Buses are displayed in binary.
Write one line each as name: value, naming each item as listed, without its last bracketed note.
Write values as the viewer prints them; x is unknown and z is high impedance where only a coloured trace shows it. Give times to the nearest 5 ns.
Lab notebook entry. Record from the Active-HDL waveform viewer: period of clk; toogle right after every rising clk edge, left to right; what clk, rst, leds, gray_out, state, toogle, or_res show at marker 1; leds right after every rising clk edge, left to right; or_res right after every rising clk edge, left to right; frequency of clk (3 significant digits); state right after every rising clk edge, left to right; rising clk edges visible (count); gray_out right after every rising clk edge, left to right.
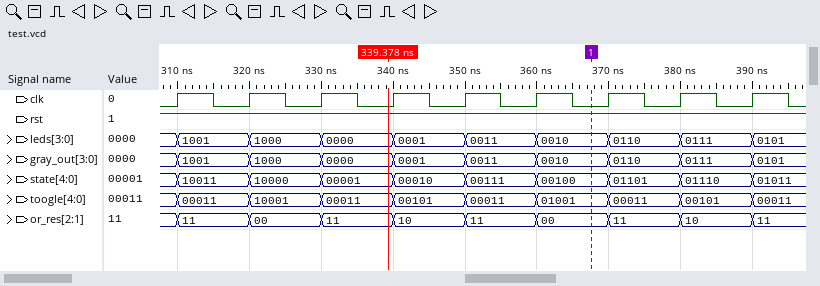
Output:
period of clk: 10 ns
toogle right after every rising clk edge, left to right: 00011, 10001, 00011, 00101, 00011, 01001, 00011, 00101, 00011
what clk, rst, leds, gray_out, state, toogle, or_res show at marker 1: clk=0, rst=1, leds=0010, gray_out=0010, state=00100, toogle=01001, or_res=00
leds right after every rising clk edge, left to right: 1001, 1000, 0000, 0001, 0011, 0010, 0110, 0111, 0101
or_res right after every rising clk edge, left to right: 11, 00, 11, 10, 11, 00, 11, 10, 11
frequency of clk: 100 MHz
state right after every rising clk edge, left to right: 10011, 10000, 00001, 00010, 00111, 00100, 01101, 01110, 01011
rising clk edges visible: 9
gray_out right after every rising clk edge, left to right: 1001, 1000, 0000, 0001, 0011, 0010, 0110, 0111, 0101
